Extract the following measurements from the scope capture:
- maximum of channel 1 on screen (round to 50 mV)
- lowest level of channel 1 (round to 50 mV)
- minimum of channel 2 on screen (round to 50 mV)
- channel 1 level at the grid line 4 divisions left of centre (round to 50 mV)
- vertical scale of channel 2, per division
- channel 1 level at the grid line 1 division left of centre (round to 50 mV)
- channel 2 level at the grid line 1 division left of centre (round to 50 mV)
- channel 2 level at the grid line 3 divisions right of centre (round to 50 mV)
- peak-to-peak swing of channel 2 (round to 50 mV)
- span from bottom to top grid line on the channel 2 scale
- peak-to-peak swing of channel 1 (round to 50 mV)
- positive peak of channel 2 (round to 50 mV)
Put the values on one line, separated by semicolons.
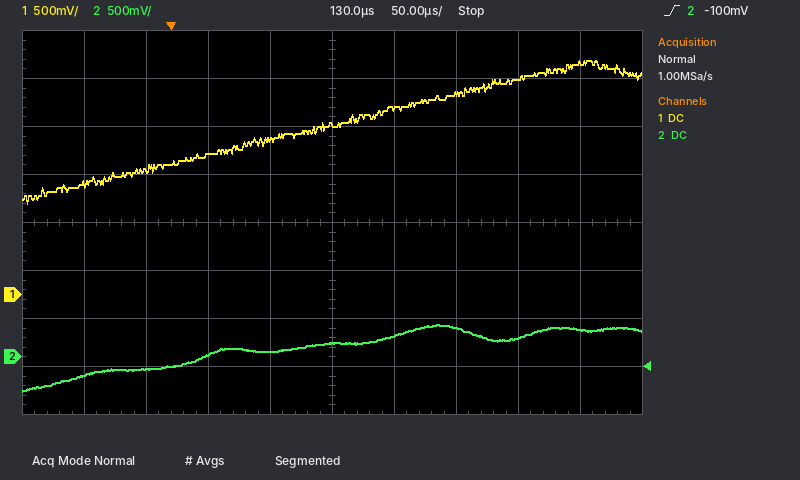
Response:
2.45 V; 950 mV; -350 mV; 1.15 V; 500 mV; 1.60 V; 50 mV; 200 mV; 700 mV; 4 V; 1.50 V; 350 mV
